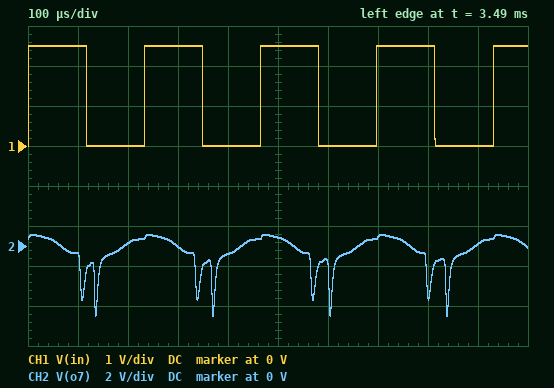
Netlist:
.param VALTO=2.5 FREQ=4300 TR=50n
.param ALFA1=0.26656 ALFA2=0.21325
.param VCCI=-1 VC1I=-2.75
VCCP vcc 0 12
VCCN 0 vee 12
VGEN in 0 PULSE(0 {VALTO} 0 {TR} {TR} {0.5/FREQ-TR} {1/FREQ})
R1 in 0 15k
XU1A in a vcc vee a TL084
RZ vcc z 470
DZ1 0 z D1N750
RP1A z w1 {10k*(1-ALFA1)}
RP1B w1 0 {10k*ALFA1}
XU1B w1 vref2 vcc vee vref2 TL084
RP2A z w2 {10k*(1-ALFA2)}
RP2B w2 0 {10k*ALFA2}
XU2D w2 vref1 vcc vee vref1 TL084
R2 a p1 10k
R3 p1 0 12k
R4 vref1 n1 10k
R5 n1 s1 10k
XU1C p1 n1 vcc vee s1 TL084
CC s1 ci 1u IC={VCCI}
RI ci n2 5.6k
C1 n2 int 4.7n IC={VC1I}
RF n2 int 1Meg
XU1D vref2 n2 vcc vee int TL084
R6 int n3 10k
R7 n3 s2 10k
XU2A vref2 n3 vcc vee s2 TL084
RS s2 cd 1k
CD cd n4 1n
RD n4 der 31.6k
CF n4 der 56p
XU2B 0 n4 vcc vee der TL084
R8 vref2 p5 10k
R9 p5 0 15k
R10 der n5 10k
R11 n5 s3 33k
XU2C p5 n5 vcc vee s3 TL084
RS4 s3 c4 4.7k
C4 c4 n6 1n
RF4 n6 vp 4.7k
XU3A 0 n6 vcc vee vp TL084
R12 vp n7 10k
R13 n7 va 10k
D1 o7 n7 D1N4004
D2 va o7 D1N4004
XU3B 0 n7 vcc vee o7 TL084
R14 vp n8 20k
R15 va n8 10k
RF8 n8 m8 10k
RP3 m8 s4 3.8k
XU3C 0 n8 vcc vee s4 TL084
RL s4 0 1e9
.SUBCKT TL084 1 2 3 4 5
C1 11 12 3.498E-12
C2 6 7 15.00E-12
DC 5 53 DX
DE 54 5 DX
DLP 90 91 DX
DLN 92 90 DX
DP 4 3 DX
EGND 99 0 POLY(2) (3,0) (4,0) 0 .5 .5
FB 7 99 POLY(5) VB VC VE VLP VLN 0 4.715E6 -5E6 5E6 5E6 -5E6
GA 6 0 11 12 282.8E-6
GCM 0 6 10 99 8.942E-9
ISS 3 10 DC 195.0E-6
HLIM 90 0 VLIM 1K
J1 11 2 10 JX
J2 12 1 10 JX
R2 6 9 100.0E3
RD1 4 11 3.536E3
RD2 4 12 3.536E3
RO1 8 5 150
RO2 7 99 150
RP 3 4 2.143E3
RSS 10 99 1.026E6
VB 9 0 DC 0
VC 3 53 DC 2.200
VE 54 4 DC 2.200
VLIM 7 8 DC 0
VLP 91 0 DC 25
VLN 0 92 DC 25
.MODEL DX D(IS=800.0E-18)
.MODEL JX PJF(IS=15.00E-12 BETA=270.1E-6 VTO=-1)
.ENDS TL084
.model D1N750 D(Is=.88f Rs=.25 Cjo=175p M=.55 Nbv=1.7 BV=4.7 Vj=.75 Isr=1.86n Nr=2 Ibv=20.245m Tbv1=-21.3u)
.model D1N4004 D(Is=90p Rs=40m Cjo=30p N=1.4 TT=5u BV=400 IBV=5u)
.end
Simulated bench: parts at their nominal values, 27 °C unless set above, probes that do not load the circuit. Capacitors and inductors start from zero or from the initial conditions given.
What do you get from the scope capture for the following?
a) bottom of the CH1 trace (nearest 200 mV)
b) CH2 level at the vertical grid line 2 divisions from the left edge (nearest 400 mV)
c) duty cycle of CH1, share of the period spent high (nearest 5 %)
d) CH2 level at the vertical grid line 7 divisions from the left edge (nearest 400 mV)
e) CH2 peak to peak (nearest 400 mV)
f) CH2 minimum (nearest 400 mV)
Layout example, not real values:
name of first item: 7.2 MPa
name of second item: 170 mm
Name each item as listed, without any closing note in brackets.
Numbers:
bottom of the CH1 trace: 0 V
CH2 level at the vertical grid line 2 divisions from the left edge: 0 V
duty cycle of CH1, share of the period spent high: 50 %
CH2 level at the vertical grid line 7 divisions from the left edge: 400 mV
CH2 peak to peak: 4.0 V
CH2 minimum: -3.6 V
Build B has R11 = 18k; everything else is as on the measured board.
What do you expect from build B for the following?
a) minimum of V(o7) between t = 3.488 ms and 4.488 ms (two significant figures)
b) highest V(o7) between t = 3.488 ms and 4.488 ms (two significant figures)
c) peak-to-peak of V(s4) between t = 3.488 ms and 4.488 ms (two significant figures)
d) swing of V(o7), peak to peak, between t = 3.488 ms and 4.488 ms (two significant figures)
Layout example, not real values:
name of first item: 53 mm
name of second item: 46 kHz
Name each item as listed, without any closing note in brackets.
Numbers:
minimum of V(o7) between t = 3.488 ms and 4.488 ms: -2.1 V
highest V(o7) between t = 3.488 ms and 4.488 ms: 530 mV
peak-to-peak of V(s4) between t = 3.488 ms and 4.488 ms: 2.2 V
swing of V(o7), peak to peak, between t = 3.488 ms and 4.488 ms: 2.7 V
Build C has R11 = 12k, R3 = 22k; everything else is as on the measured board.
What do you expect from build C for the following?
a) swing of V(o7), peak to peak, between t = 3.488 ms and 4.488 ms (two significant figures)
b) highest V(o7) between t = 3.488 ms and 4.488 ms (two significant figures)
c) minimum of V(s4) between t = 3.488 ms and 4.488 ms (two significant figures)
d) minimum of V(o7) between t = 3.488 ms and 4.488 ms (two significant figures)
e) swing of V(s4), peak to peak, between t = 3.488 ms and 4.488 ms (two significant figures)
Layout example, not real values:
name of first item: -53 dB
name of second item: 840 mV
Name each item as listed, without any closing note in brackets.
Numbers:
swing of V(o7), peak to peak, between t = 3.488 ms and 4.488 ms: 2.3 V
highest V(o7) between t = 3.488 ms and 4.488 ms: 520 mV
minimum of V(s4) between t = 3.488 ms and 4.488 ms: -270 mV
minimum of V(o7) between t = 3.488 ms and 4.488 ms: -1.8 V
swing of V(s4), peak to peak, between t = 3.488 ms and 4.488 ms: 2.1 V
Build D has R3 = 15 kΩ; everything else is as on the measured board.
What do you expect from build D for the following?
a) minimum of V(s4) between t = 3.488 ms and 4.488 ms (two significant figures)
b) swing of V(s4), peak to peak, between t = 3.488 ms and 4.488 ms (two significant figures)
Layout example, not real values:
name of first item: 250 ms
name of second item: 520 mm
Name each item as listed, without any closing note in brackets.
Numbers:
minimum of V(s4) between t = 3.488 ms and 4.488 ms: -190 mV
swing of V(s4), peak to peak, between t = 3.488 ms and 4.488 ms: 4.6 V
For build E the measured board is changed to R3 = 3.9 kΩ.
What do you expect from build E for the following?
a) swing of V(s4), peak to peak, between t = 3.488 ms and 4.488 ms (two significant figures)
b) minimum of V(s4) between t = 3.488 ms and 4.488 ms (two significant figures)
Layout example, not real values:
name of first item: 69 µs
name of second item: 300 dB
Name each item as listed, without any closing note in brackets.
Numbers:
swing of V(s4), peak to peak, between t = 3.488 ms and 4.488 ms: 2.5 V
minimum of V(s4) between t = 3.488 ms and 4.488 ms: -400 mV
